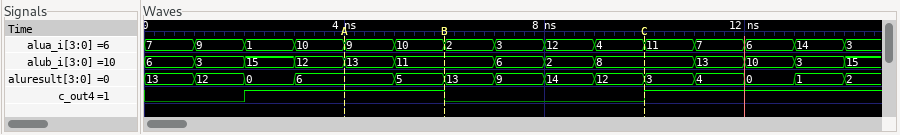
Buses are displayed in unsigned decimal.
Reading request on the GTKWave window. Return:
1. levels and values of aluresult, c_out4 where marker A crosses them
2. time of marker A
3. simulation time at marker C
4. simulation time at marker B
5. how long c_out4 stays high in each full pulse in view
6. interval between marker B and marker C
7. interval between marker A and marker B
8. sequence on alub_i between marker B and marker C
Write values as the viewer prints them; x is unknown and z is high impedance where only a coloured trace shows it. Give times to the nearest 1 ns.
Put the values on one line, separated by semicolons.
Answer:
aluresult=6, c_out4=1; 4 ns; 10 ns; 6 ns; 4 ns; 4 ns; 2 ns; 11, 6, 2, 8
